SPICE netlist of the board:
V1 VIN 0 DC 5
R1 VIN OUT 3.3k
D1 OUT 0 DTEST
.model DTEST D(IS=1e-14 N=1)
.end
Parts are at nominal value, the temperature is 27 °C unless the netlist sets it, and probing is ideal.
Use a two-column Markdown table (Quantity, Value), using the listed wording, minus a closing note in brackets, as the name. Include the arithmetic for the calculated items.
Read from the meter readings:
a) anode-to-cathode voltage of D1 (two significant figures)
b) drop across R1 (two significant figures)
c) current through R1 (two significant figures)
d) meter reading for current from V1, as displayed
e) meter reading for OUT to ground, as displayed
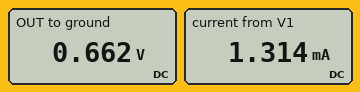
| Quantity | Value |
|---|---|
| anode-to-cathode voltage of D1 | 662 mV = 660 mV |
| drop across R1 | 5 V - 662 mV = 4.3 V |
| current through R1 | (5 V - 662 mV) / 3.3 kΩ = 1.3 mA |
| meter reading for current from V1, as displayed | 1.314 mA |
| meter reading for OUT to ground, as displayed | 0.662 V |
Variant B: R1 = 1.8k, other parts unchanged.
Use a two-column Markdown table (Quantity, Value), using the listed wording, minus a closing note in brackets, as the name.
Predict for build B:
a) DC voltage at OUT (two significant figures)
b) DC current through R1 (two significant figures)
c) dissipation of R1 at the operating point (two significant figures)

| Quantity | Value |
|---|---|
| DC voltage at OUT | 680 mV |
| DC current through R1 | 2.4 mA |
| dissipation of R1 at the operating point | 10 mW |
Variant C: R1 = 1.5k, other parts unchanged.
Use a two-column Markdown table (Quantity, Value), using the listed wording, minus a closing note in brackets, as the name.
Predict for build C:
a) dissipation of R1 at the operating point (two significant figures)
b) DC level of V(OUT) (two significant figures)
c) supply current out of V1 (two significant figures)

| Quantity | Value |
|---|---|
| dissipation of R1 at the operating point | 12 mW |
| DC level of V(OUT) | 680 mV |
| supply current out of V1 | 2.9 mA |
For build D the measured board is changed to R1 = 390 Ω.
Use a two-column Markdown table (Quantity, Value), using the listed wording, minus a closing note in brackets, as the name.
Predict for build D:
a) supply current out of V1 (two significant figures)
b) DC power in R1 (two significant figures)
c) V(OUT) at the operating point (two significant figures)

| Quantity | Value |
|---|---|
| supply current out of V1 | 11 mA |
| DC power in R1 | 47 mW |
| V(OUT) at the operating point | 720 mV |
